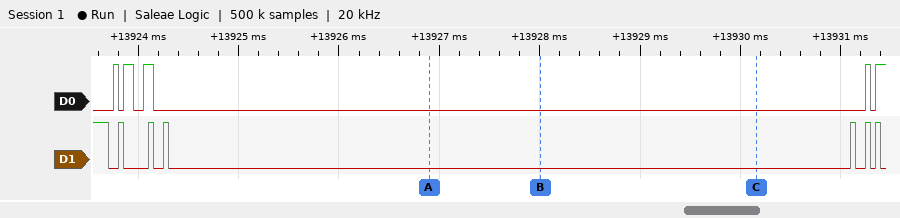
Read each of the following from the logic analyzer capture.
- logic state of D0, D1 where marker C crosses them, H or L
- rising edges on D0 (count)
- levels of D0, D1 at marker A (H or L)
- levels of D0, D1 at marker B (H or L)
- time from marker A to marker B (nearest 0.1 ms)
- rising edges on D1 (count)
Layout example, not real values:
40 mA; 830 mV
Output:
D0=L, D1=L; 5; D0=L, D1=L; D0=L, D1=L; 1.1 ms; 6
